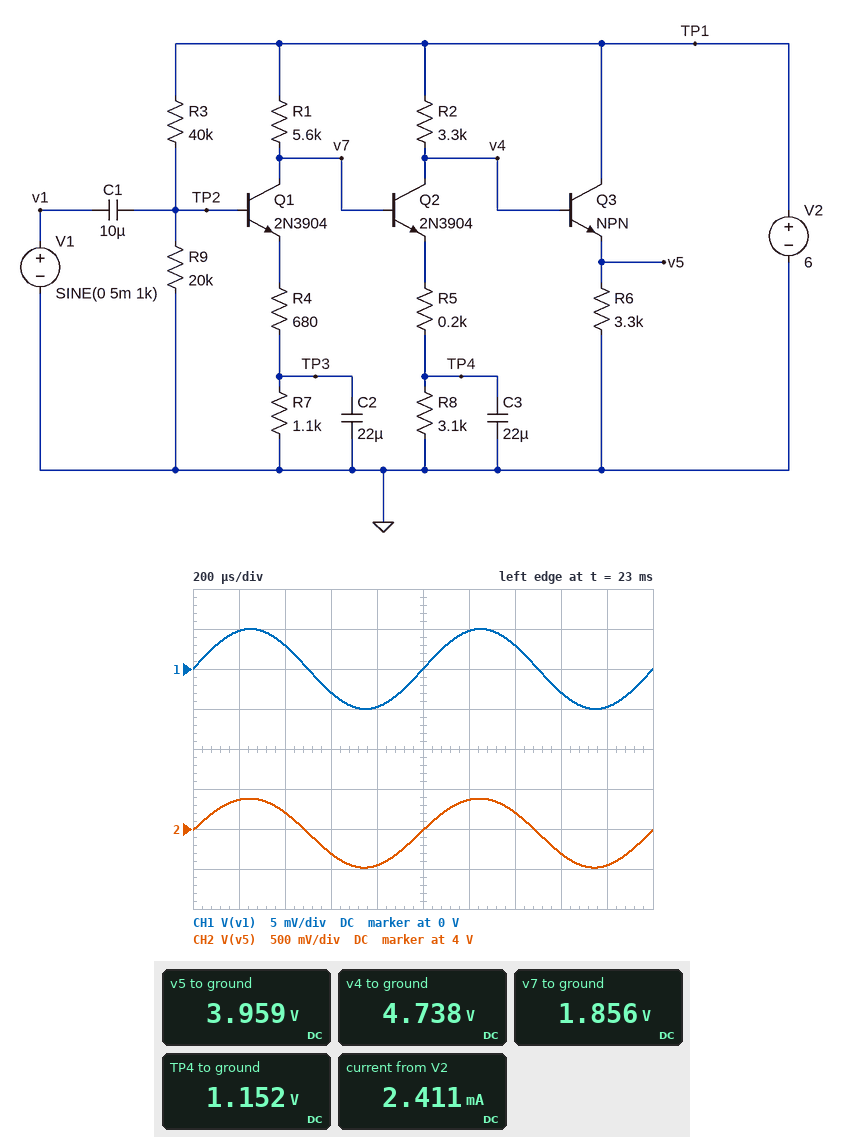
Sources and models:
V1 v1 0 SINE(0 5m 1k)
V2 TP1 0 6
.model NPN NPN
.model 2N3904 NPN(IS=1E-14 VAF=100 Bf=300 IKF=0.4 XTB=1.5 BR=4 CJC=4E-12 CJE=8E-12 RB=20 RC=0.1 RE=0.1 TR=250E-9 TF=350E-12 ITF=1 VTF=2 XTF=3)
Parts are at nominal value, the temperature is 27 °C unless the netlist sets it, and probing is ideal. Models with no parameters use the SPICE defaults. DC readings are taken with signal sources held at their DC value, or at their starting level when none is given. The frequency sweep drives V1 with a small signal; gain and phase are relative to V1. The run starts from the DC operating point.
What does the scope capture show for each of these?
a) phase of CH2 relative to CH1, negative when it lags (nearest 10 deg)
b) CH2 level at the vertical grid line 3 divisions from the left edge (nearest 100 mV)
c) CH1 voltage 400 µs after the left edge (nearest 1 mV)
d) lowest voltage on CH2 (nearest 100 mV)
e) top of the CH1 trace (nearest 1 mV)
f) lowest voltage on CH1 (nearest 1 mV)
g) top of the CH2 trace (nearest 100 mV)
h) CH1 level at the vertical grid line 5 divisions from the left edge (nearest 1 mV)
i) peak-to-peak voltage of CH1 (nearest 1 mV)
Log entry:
0 deg
3.7 V
3 mV
3.5 V
5 mV
-5 mV
4.4 V
0 V
10 mV
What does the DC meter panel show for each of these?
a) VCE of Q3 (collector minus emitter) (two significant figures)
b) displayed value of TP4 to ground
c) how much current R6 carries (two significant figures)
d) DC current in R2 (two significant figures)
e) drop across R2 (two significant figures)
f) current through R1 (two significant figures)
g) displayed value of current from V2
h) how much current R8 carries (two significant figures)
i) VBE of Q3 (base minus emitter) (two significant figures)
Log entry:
2.0 V
1.152 V
1.2 mA
380 µA
1.3 V
740 µA
2.411 mA
370 µA
780 mV
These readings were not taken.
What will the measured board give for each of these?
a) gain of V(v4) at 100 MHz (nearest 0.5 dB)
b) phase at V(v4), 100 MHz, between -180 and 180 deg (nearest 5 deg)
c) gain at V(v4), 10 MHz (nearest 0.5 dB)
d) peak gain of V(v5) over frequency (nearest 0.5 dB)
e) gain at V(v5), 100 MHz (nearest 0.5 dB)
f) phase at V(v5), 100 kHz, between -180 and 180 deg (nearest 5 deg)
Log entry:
3.0 dB
120 deg
16.5 dB
39.0 dB
3.0 dB
-10 deg
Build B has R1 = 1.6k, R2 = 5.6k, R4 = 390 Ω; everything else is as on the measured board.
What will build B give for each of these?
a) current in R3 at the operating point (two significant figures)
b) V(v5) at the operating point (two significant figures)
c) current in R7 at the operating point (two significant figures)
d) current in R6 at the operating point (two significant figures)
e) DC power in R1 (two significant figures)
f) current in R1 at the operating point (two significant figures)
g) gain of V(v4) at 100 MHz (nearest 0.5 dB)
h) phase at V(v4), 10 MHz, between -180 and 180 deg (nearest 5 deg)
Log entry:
100 µA
2.4 V
880 µA
730 µA
2.9 mW
1.3 mA
-5.5 dB
170 deg
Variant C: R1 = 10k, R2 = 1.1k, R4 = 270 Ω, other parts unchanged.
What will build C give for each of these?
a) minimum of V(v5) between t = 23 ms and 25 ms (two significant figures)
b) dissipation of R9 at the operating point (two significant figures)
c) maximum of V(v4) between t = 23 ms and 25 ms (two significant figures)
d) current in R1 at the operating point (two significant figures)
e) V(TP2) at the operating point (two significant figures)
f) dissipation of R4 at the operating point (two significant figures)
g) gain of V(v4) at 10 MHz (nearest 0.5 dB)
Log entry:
5.1 V
100 µW
5.9 V
520 µA
1.4 V
85 µW
5.0 dB
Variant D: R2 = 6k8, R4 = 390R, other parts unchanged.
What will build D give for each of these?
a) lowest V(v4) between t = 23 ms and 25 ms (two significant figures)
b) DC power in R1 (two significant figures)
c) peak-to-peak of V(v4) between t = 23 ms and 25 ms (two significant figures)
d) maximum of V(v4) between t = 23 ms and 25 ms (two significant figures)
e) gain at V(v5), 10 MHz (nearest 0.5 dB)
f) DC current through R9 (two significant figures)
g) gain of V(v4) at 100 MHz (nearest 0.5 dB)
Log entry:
3.7 V
3.9 mW
1.2 V
4.9 V
21.5 dB
95 µA
6.0 dB
